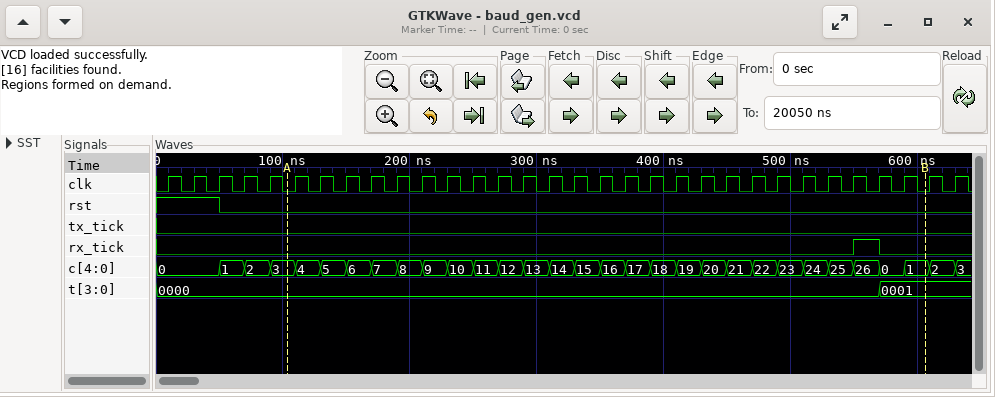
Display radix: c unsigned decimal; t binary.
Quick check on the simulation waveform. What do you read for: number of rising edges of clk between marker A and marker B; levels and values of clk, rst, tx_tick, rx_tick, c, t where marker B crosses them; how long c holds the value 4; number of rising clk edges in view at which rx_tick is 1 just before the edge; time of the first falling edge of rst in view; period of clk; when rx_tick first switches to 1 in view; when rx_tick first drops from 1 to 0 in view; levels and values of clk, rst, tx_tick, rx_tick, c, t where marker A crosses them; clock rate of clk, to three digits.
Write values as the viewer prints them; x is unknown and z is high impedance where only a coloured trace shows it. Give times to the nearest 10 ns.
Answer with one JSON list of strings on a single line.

["25", "clk=0, rst=0, tx_tick=0, rx_tick=0, c=1, t=0001", "20 ns", "1", "50 ns", "20 ns", "550 ns", "570 ns", "clk=0, rst=0, tx_tick=0, rx_tick=0, c=3, t=0000", "50.0 MHz"]
